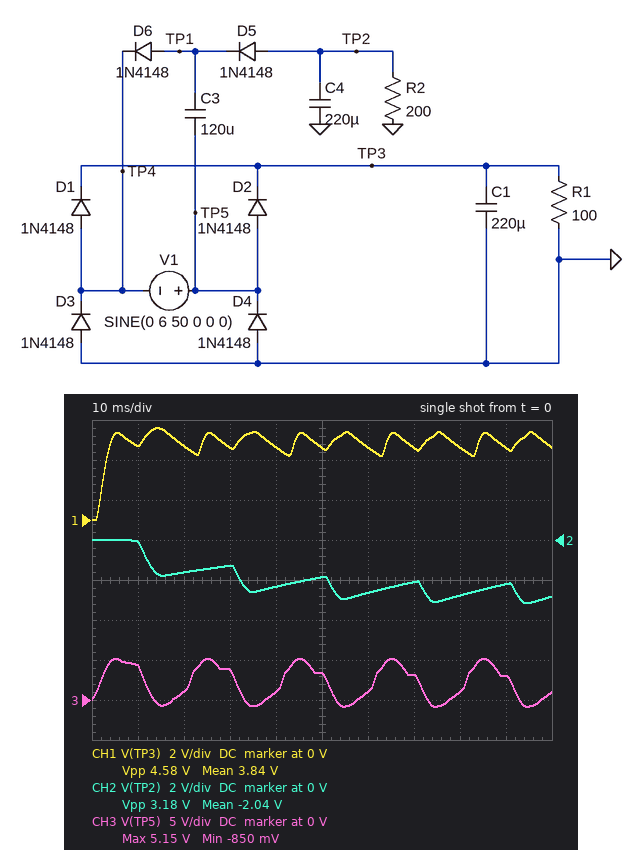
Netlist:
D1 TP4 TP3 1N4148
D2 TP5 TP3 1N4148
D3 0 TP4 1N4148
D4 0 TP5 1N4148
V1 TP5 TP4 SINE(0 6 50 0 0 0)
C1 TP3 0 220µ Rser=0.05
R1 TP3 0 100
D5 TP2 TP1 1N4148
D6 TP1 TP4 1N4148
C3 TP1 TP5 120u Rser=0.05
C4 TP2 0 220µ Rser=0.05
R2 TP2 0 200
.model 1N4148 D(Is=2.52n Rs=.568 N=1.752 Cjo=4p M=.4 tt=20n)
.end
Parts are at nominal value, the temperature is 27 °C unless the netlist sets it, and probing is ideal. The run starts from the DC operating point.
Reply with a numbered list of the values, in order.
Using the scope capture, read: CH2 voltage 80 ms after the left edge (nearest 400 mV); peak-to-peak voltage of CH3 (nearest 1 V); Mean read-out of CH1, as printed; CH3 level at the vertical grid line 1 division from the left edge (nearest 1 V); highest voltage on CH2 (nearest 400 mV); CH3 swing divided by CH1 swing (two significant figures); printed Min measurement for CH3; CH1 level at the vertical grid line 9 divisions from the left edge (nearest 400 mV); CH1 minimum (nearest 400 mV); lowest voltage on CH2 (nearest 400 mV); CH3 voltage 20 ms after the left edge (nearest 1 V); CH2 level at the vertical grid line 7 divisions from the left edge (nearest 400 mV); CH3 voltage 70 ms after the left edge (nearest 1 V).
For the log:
1. -2.8 V
2. 6 V
3. 3.84 V
4. 4 V
5. 0 V
6. 1.3
7. -850 mV
8. 3.6 V
9. 0 V
10. -3.2 V
11. 1 V
12. -2.0 V
13. 3 V
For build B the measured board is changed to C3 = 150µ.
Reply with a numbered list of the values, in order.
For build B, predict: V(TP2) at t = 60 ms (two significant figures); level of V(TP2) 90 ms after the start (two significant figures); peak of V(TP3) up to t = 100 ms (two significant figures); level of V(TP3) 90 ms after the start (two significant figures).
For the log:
1. -2.9 V
2. -2.4 V
3. 4.8 V
4. 3.6 V
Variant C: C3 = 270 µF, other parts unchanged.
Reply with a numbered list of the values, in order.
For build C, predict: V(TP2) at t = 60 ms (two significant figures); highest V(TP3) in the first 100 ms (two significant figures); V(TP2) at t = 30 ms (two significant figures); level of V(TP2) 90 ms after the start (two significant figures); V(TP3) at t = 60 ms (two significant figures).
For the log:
1. -3.5 V
2. 5.2 V
3. -1.8 V
4. -2.9 V
5. 3.7 V
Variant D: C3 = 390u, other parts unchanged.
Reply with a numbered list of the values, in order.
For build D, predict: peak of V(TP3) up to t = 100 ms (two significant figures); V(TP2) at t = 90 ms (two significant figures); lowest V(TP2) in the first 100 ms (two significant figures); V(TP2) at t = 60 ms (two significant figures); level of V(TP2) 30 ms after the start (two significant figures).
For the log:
1. 5.4 V
2. -3.1 V
3. -4.3 V
4. -3.8 V
5. -2.0 V
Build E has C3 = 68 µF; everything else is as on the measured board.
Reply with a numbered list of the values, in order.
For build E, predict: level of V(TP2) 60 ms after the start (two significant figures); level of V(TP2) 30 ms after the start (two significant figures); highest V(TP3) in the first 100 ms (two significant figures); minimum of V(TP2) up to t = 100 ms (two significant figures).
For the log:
1. -1.9 V
2. -880 mV
3. 4.4 V
4. -2.4 V
